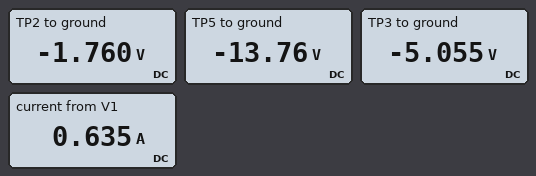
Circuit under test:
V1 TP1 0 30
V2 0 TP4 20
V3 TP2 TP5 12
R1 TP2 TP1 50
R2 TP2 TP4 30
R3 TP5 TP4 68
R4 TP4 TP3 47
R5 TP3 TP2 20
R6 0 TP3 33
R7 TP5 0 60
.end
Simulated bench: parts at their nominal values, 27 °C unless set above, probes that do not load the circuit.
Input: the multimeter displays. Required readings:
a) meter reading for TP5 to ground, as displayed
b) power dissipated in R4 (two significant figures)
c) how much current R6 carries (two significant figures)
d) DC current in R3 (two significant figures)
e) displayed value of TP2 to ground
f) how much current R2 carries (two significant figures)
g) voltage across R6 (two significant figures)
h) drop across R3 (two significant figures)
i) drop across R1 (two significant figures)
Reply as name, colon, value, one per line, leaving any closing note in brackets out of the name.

meter reading for TP5 to ground, as displayed: -13.76 V
power dissipated in R4: 4.8 W
how much current R6 carries: 150 mA
DC current in R3: 92 mA
displayed value of TP2 to ground: -1.760 V
how much current R2 carries: 610 mA
voltage across R6: 5.1 V
drop across R3: 6.2 V
drop across R1: 32 V
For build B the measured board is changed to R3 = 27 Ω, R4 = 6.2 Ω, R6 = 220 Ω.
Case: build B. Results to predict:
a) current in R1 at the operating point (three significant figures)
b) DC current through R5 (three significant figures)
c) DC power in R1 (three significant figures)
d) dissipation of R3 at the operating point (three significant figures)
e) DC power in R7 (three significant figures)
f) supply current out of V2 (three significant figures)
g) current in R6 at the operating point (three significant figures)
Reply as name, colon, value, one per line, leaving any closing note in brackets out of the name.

current in R1 at the operating point: 725 mA
DC current through R5: 507 mA
DC power in R1: 26.3 W
dissipation of R3 at the operating point: 112 mW
DC power in R7: 5.56 W
supply current out of V2: 1.10 A
current in R6 at the operating point: 74.5 mA
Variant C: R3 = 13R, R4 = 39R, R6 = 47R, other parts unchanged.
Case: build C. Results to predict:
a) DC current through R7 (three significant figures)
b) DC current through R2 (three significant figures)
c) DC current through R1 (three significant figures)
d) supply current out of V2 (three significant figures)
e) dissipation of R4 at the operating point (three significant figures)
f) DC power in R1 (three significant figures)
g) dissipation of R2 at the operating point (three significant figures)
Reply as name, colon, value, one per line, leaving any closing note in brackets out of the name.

DC current through R7: 273 mA
DC current through R2: 521 mA
DC current through R1: 687 mA
supply current out of V2: 1.12 A
dissipation of R4 at the operating point: 3.98 W
DC power in R1: 23.6 W
dissipation of R2 at the operating point: 8.15 W
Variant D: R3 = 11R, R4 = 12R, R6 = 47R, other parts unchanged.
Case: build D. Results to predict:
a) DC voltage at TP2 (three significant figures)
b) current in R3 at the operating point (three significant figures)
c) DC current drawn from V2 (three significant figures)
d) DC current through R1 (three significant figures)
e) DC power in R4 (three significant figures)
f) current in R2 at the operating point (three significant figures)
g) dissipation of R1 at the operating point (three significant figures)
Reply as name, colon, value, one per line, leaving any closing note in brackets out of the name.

DC voltage at TP2: -5.82 V
current in R3 at the operating point: 198 mA
DC current drawn from V2: 1.28 A
DC current through R1: 716 mA
DC power in R4: 4.49 W
current in R2 at the operating point: 473 mA
dissipation of R1 at the operating point: 25.7 W
